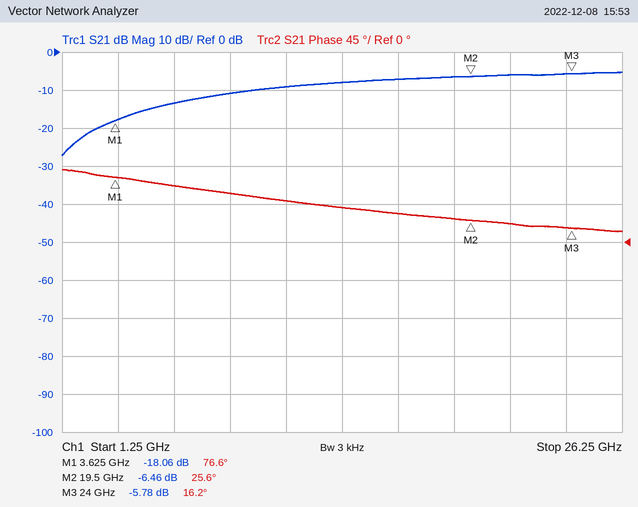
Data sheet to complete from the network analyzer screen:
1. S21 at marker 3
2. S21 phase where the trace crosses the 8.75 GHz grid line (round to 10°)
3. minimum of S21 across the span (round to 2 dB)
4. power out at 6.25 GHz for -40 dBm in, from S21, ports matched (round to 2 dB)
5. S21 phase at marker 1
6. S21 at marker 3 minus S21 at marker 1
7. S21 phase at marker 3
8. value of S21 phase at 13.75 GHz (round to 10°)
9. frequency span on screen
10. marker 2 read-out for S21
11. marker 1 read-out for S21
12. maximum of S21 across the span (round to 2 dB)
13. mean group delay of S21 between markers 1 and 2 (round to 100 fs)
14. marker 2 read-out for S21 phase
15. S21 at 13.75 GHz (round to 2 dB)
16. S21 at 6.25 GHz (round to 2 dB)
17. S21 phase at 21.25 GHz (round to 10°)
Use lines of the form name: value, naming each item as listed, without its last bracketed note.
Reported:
S21 at marker 3: -5.78 dB
S21 phase where the trace crosses the 8.75 GHz grid line: 60°
minimum of S21 across the span: -28 dB
power out at 6.25 GHz for -40 dBm in, from S21, ports matched: -54 dBm
S21 phase at marker 1: 76.6°
S21 at marker 3 minus S21 at marker 1: 12.28 dB
S21 phase at marker 3: 16.2°
value of S21 phase at 13.75 GHz: 40°
frequency span on screen: 25 GHz
marker 2 read-out for S21: -6.46 dB
marker 1 read-out for S21: -18.06 dB
maximum of S21 across the span: -6 dB
mean group delay of S21 between markers 1 and 2: 8.9 ps
marker 2 read-out for S21 phase: 25.6°
S21 at 13.75 GHz: -8 dB
S21 at 6.25 GHz: -14 dB
S21 phase at 21.25 GHz: 20°
